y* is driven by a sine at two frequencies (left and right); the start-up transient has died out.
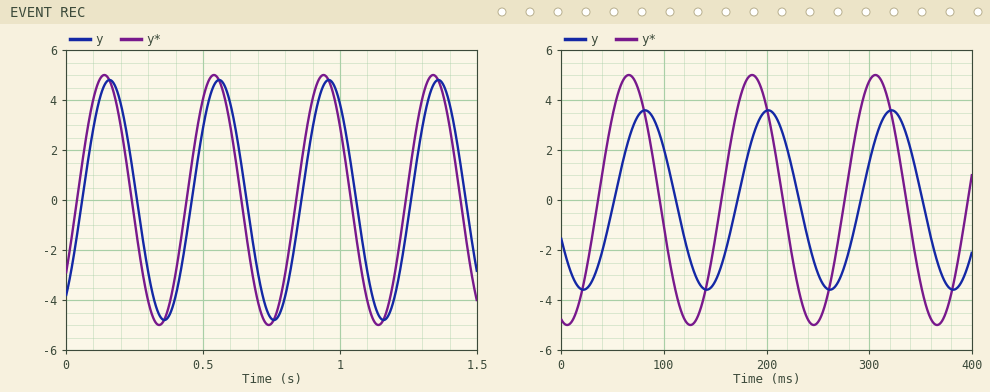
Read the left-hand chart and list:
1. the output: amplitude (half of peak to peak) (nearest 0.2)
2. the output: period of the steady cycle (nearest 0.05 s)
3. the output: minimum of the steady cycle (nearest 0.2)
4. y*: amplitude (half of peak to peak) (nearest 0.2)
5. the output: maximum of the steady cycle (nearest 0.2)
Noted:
4.8
0.40 s
-4.8
5.0
4.8
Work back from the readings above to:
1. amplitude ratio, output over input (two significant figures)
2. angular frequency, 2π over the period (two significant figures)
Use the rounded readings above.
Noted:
0.96
16 rad/s
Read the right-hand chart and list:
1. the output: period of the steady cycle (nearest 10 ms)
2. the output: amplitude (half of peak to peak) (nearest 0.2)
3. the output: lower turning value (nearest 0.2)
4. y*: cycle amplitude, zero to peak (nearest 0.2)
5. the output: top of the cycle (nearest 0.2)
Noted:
120 ms
3.6
-3.6
5.0
3.6
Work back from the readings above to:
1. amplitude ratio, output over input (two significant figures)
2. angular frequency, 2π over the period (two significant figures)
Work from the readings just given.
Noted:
0.72
0.052 rad/ms
